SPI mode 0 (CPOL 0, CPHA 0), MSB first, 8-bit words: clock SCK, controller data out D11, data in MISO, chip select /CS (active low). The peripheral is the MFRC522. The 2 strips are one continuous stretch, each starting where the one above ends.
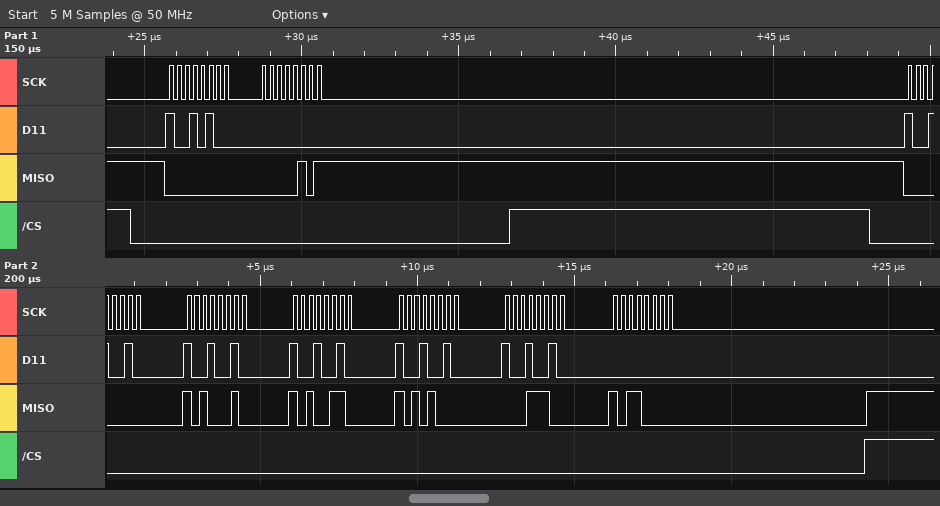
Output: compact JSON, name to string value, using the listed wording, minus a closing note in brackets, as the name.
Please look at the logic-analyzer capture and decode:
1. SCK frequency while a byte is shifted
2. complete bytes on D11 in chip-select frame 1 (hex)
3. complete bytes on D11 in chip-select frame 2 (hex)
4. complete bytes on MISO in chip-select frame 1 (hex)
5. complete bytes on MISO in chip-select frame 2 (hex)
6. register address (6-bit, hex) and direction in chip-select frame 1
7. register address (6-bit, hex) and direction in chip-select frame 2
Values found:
{"SCK frequency while a byte is shifted": "4 MHz", "complete bytes on D11 in chip-select frame 1": "0x94 0x00", "complete bytes on D11 in chip-select frame 2": "0x92 0x92 0x92 0x92 0x92 0x00", "complete bytes on MISO in chip-select frame 1": "0x00 0x05", "complete bytes on MISO in chip-select frame 2": "0x00 0xA2 0xA6 0xA8 0x1C 0xB0", "register address (6-bit, hex) and direction in chip-select frame 1": "0x0A read", "register address (6-bit, hex) and direction in chip-select frame 2": "0x09 read"}
